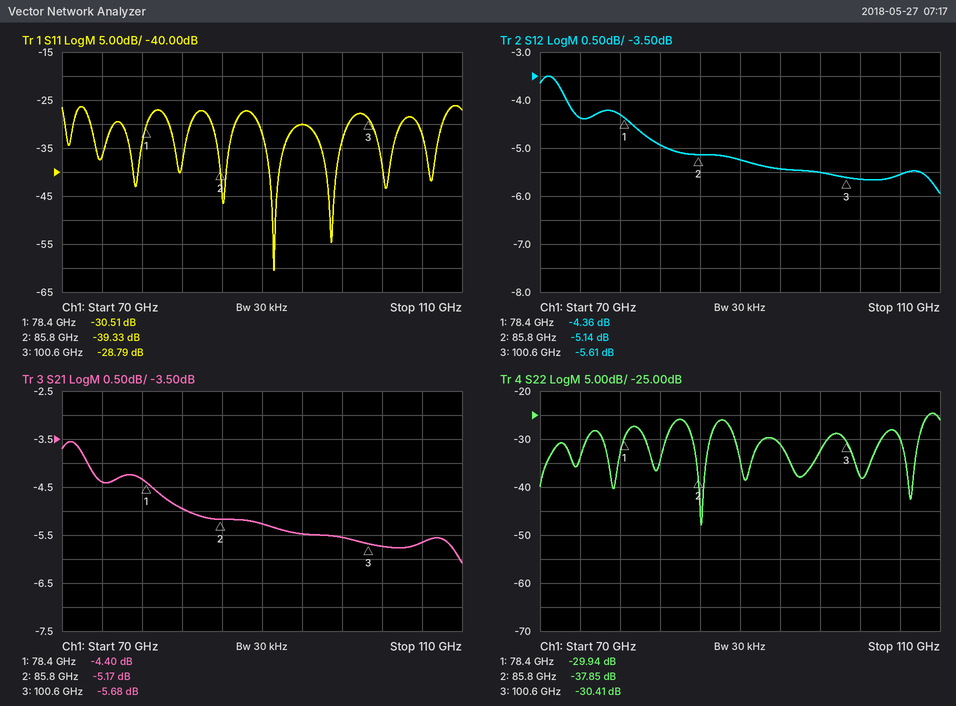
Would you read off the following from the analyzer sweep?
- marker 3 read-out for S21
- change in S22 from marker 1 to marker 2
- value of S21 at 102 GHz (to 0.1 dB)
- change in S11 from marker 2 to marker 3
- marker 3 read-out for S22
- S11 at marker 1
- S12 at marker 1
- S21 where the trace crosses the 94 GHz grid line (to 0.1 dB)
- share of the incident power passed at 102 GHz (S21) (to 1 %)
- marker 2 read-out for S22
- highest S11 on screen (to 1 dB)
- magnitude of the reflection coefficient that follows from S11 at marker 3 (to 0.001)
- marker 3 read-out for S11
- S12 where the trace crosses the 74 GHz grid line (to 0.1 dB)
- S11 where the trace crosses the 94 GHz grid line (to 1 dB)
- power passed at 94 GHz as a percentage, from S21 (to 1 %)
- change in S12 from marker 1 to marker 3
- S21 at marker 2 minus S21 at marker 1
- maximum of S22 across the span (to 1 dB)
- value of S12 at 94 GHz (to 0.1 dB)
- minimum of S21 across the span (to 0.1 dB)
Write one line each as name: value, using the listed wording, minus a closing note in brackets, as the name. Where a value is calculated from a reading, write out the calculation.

marker 3 read-out for S21: -5.68 dB
change in S22 from marker 1 to marker 2: -37.85 − (-29.94) = -7.91 dB
value of S21 at 102 GHz: -5.7 dB
change in S11 from marker 2 to marker 3: -28.79 − (-39.33) = 10.54 dB
marker 3 read-out for S22: -30.41 dB
S11 at marker 1: -30.51 dB
S12 at marker 1: -4.36 dB
S21 where the trace crosses the 94 GHz grid line: -5.5 dB
share of the incident power passed at 102 GHz (S21): 10^(-5.7/10) ≈ 27 %
marker 2 read-out for S22: -37.85 dB
highest S11 on screen: -26 dB
magnitude of the reflection coefficient that follows from S11 at marker 3: 10^(-28.79/20) ≈ 0.036
marker 3 read-out for S11: -28.79 dB
S12 where the trace crosses the 74 GHz grid line: -4.4 dB
S11 where the trace crosses the 94 GHz grid line: -30 dB
power passed at 94 GHz as a percentage, from S21: 10^(-5.5/10) ≈ 28 %
change in S12 from marker 1 to marker 3: -5.61 − (-4.36) = -1.25 dB
S21 at marker 2 minus S21 at marker 1: -5.17 − (-4.4) = -0.77 dB
maximum of S22 across the span: -25 dB
value of S12 at 94 GHz: -5.4 dB
minimum of S21 across the span: -6.1 dB
